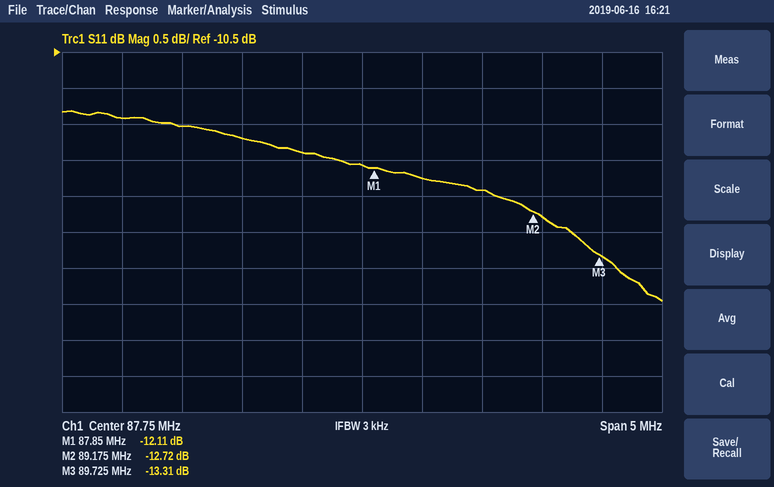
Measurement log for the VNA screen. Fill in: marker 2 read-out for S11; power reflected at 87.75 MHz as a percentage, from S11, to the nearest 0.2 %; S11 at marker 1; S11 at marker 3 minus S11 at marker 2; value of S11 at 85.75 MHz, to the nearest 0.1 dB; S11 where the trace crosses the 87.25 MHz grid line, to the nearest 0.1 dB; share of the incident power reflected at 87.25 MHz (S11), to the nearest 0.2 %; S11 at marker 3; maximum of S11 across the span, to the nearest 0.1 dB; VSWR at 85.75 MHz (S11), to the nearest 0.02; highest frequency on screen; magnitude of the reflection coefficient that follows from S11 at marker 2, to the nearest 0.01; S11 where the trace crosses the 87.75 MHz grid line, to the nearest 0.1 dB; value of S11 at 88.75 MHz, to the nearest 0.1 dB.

-12.72 dB
6.2 %
-12.11 dB
-0.59 dB
-11.4 dB
-11.9 dB
6.4 %
-13.31 dB
-11.3 dB
1.74
90.25 MHz
0.23
-12.1 dB
-12.4 dB
